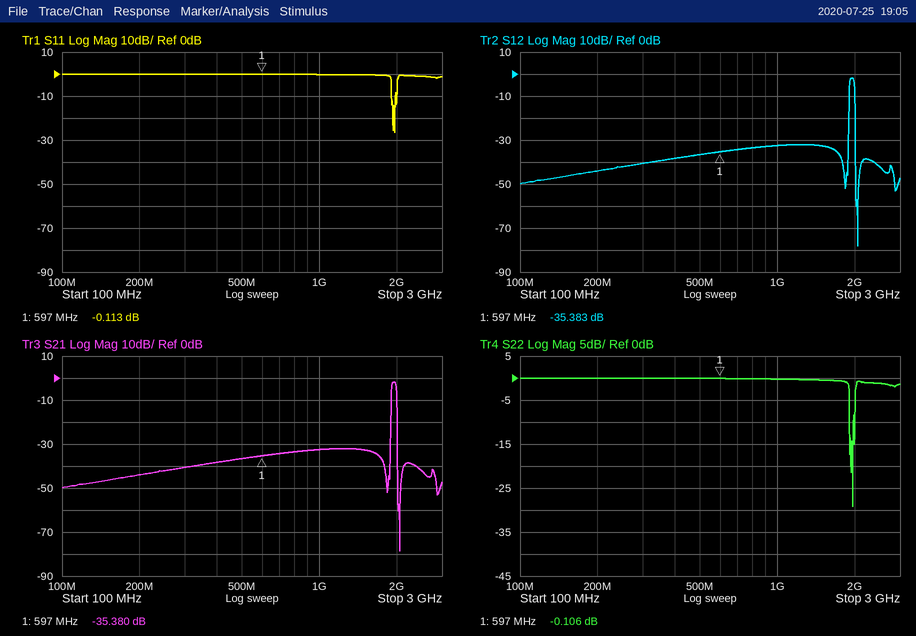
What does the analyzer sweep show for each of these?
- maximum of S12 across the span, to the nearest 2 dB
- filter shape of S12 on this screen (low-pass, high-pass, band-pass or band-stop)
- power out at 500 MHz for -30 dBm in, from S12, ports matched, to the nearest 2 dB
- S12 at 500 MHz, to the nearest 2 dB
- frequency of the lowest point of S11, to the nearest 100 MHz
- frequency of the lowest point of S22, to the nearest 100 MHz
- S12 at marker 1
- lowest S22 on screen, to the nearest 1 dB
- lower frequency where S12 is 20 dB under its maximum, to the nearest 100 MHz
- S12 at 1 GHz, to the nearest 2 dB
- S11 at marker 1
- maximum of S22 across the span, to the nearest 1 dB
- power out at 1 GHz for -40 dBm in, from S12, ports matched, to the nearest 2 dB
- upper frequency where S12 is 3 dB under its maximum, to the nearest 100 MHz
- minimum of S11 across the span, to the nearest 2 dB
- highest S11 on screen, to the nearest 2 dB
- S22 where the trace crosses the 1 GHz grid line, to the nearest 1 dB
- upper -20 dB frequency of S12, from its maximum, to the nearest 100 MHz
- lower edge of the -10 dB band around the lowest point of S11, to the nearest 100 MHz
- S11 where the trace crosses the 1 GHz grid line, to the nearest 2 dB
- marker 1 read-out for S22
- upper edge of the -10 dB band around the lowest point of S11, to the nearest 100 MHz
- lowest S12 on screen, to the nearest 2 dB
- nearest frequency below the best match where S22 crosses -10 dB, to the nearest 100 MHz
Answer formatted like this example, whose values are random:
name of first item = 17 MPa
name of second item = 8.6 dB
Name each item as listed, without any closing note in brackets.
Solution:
maximum of S12 across the span, to the nearest 2 dB = -2 dB
filter shape of S12 on this screen = band-pass
power out at 500 MHz for -30 dBm in, from S12, ports matched, to the nearest 2 dB = -66 dBm
S12 at 500 MHz, to the nearest 2 dB = -36 dB
frequency of the lowest point of S11, to the nearest 100 MHz = 2.0 GHz
frequency of the lowest point of S22, to the nearest 100 MHz = 2.0 GHz
S12 at marker 1 = -35.383 dB
lowest S22 on screen, to the nearest 1 dB = -29 dB
lower frequency where S12 is 20 dB under its maximum, to the nearest 100 MHz = 1.9 GHz
S12 at 1 GHz, to the nearest 2 dB = -32 dB
S11 at marker 1 = -0.113 dB
maximum of S22 across the span, to the nearest 1 dB = 0 dB
power out at 1 GHz for -40 dBm in, from S12, ports matched, to the nearest 2 dB = -72 dBm
upper frequency where S12 is 3 dB under its maximum, to the nearest 100 MHz = 2.0 GHz
minimum of S11 across the span, to the nearest 2 dB = -26 dB
highest S11 on screen, to the nearest 2 dB = 0 dB
S22 where the trace crosses the 1 GHz grid line, to the nearest 1 dB = 0 dB
upper -20 dB frequency of S12, from its maximum, to the nearest 100 MHz = 2.0 GHz
lower edge of the -10 dB band around the lowest point of S11, to the nearest 100 MHz = 1.9 GHz
S11 where the trace crosses the 1 GHz grid line, to the nearest 2 dB = 0 dB
marker 1 read-out for S22 = -0.106 dB
upper edge of the -10 dB band around the lowest point of S11, to the nearest 100 MHz = 2.0 GHz
lowest S12 on screen, to the nearest 2 dB = -78 dB
nearest frequency below the best match where S22 crosses -10 dB, to the nearest 100 MHz = 1.9 GHz
